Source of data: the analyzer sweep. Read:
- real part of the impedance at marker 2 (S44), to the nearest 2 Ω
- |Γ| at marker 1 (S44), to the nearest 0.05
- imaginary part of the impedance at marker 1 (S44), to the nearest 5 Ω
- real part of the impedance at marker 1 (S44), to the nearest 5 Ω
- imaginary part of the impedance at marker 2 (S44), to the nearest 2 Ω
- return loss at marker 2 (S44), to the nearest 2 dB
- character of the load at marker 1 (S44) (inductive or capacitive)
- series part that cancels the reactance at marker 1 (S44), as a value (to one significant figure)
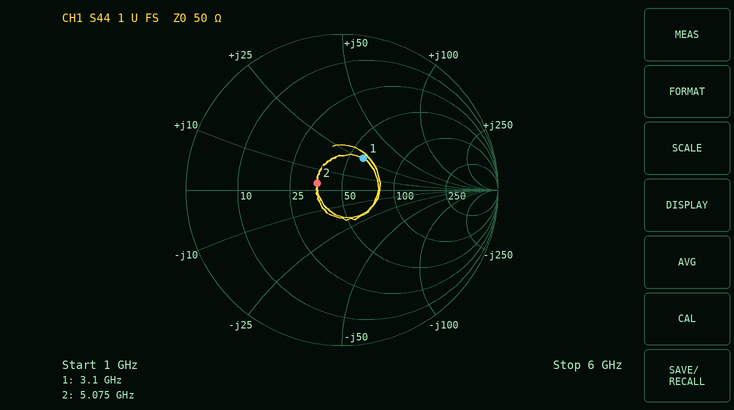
36 Ω
0.25
+25 Ω
60 Ω
+4 Ω
16 dB
inductive
2 pF
